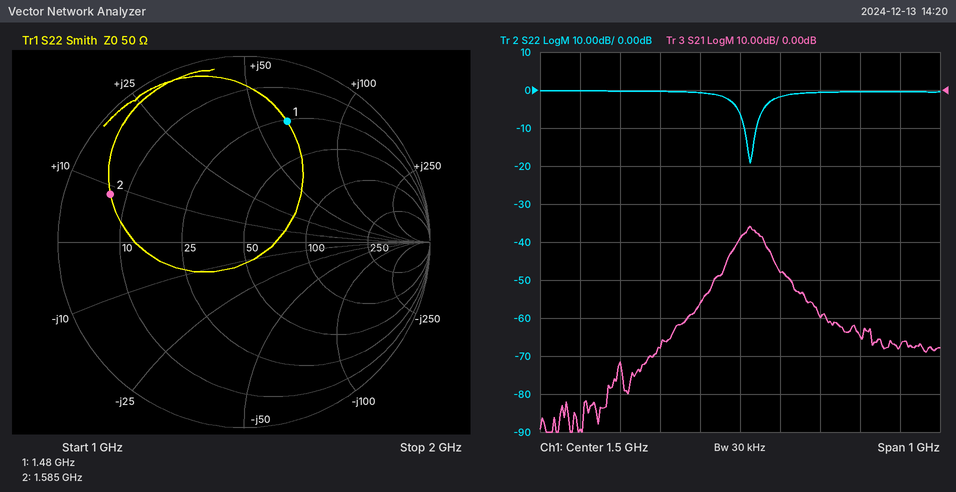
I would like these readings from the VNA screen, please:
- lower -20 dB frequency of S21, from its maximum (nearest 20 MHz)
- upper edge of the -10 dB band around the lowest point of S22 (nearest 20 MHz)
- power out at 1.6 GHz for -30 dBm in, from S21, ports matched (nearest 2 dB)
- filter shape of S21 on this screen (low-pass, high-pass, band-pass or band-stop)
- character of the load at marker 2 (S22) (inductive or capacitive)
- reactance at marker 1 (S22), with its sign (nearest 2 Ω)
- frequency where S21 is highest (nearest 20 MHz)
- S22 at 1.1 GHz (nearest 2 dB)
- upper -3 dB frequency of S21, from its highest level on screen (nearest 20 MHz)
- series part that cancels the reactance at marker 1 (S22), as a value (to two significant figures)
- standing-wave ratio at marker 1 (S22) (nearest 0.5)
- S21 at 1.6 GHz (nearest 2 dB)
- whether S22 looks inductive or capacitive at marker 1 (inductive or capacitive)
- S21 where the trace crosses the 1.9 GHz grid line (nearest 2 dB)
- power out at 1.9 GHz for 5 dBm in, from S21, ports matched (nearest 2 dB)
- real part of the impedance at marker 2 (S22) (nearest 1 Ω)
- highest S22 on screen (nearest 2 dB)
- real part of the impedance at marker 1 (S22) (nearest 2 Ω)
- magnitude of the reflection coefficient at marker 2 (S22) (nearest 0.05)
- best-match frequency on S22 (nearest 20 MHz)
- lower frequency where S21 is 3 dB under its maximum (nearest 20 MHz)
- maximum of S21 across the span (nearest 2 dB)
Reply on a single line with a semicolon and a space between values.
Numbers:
1.40 GHz; 1.54 GHz; -78 dBm; band-pass; inductive; +64 Ω; 1.52 GHz; 0 dB; 1.56 GHz; 1.7 pF; 5.5; -48 dB; inductive; -68 dB; -62 dBm; 7 Ω; 0 dB; 26 Ω; 0.75; 1.52 GHz; 1.50 GHz; -36 dB
